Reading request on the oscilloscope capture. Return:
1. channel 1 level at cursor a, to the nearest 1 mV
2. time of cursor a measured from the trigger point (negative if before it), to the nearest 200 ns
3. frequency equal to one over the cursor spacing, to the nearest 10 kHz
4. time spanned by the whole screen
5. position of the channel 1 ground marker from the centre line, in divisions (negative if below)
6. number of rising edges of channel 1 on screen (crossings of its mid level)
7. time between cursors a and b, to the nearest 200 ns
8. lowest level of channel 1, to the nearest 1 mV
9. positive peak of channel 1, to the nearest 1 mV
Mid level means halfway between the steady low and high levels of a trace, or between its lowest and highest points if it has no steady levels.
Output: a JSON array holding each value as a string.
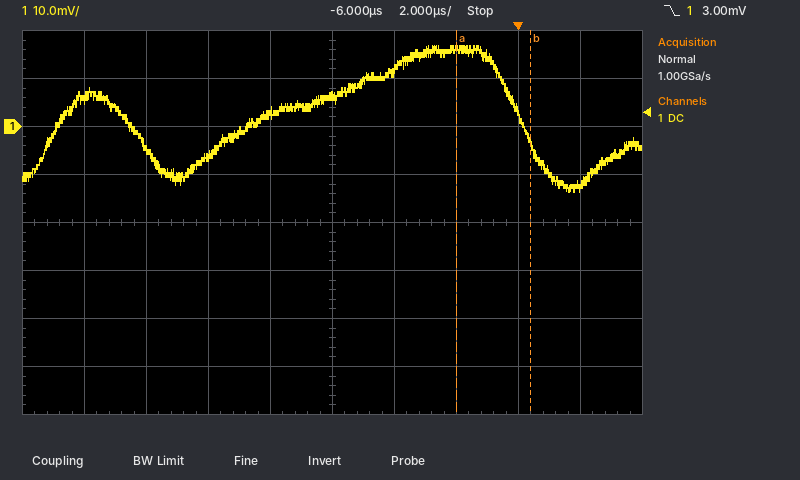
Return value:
["16 mV", "-2.0 µs", "420 kHz", "20 µs", "+2.0 div", "2", "2.4 µs", "-14 mV", "17 mV"]
